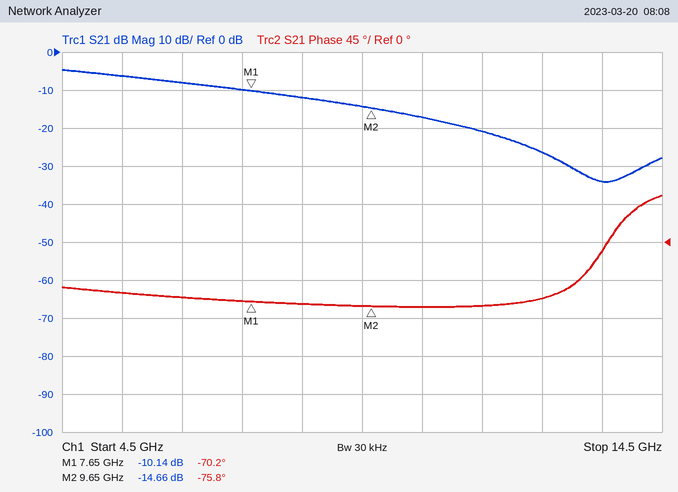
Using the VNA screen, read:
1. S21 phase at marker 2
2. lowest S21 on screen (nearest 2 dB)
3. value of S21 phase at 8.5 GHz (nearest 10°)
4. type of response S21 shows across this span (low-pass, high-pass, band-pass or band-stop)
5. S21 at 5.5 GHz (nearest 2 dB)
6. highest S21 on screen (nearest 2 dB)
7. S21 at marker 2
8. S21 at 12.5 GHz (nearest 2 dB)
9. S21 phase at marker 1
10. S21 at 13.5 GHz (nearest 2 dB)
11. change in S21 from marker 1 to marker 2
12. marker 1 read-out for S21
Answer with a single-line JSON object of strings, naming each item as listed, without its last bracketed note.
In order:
{"S21 phase at marker 2": "-75.8°", "lowest S21 on screen": "-34 dB", "value of S21 phase at 8.5 GHz": "-70°", "type of response S21 shows across this span": "low-pass", "S21 at 5.5 GHz": "-6 dB", "highest S21 on screen": "-4 dB", "S21 at marker 2": "-14.66 dB", "S21 at 12.5 GHz": "-26 dB", "S21 phase at marker 1": "-70.2°", "S21 at 13.5 GHz": "-34 dB", "change in S21 from marker 1 to marker 2": "-4.52 dB", "marker 1 read-out for S21": "-10.14 dB"}
